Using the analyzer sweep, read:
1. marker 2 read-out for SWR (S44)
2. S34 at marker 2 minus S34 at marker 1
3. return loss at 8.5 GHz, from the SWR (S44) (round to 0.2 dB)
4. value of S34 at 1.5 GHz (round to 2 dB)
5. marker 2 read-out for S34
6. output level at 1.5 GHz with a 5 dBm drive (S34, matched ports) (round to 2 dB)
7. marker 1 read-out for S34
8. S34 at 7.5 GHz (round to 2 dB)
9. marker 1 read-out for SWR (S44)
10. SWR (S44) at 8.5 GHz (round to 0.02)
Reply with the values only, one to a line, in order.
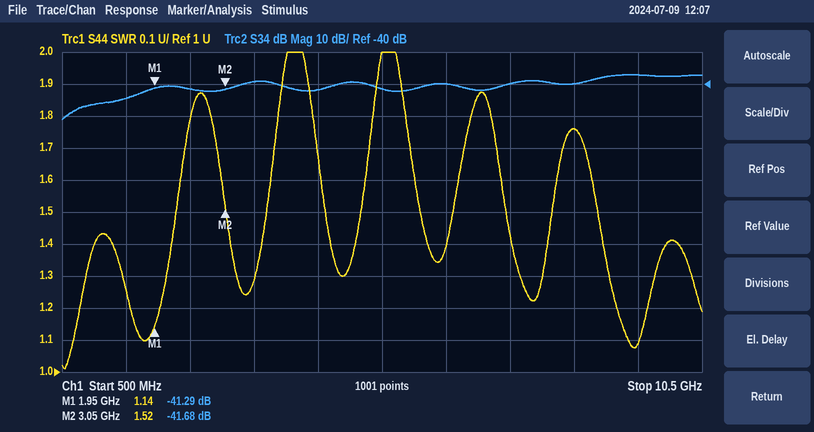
1.52
-0.39 dB
11.2 dB
-44 dB
-41.68 dB
-40 dBm
-41.29 dB
-40 dB
1.14
1.76
